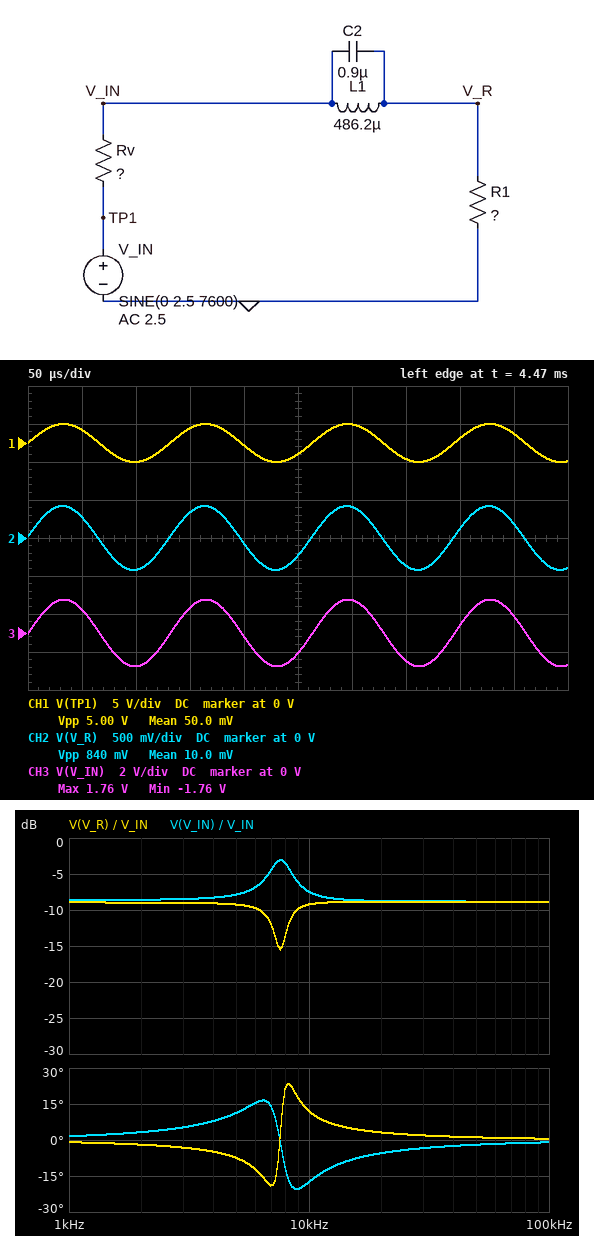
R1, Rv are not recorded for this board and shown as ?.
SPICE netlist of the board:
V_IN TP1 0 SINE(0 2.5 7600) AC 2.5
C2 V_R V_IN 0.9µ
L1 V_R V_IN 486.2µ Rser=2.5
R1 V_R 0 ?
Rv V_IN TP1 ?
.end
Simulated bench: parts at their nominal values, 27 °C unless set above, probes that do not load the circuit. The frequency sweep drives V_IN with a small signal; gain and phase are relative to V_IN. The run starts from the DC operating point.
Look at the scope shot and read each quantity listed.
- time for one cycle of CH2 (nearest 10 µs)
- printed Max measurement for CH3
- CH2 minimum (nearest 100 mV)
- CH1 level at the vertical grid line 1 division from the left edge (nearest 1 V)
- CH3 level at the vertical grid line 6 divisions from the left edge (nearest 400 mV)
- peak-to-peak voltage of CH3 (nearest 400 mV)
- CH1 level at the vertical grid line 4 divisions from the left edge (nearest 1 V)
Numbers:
130 µs
1.76 V
-400 mV
2 V
1.6 V
3.6 V
0 V
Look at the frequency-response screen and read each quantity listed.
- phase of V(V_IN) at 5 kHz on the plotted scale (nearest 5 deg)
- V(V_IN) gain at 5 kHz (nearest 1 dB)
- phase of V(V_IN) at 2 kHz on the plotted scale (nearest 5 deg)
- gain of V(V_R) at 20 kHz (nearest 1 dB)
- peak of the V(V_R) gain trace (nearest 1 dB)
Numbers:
10 deg
-8 dB
5 deg
-9 dB
-9 dB
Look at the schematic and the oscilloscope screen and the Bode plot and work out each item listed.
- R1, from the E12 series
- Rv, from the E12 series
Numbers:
68 Ω
120 Ω
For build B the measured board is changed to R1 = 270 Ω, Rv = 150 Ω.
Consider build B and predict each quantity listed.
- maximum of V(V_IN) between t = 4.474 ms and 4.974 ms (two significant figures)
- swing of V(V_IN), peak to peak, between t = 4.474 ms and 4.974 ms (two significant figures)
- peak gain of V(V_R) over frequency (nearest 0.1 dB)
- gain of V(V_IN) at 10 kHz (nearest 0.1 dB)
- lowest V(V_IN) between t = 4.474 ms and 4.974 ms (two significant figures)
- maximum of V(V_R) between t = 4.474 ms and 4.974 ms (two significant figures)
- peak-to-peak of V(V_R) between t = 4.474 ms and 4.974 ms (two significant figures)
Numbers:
1.9 V
3.8 V
-3.8 dB
-3.7 dB
-1.9 V
1.1 V
2.1 V
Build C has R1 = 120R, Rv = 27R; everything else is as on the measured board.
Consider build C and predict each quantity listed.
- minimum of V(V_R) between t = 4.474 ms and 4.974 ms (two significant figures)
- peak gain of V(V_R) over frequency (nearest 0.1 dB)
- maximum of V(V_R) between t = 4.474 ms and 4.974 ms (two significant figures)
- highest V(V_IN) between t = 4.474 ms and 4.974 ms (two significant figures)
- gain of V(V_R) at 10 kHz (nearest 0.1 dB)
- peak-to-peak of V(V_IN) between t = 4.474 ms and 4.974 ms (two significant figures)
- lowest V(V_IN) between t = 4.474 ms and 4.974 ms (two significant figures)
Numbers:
-820 mV
-1.8 dB
820 mV
2.3 V
-2.3 dB
4.6 V
-2.3 V
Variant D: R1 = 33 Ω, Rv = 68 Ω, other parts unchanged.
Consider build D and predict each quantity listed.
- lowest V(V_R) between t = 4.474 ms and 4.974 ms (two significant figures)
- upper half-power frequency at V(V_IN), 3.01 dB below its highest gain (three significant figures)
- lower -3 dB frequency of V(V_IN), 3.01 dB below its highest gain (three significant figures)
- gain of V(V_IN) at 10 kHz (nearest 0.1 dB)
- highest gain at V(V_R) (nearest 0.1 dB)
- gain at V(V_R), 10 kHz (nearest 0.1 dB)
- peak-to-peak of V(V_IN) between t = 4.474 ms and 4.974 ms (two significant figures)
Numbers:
-260 mV
9.35 kHz
6.17 kHz
-6.2 dB
-9.7 dB
-10.7 dB
3.9 V
